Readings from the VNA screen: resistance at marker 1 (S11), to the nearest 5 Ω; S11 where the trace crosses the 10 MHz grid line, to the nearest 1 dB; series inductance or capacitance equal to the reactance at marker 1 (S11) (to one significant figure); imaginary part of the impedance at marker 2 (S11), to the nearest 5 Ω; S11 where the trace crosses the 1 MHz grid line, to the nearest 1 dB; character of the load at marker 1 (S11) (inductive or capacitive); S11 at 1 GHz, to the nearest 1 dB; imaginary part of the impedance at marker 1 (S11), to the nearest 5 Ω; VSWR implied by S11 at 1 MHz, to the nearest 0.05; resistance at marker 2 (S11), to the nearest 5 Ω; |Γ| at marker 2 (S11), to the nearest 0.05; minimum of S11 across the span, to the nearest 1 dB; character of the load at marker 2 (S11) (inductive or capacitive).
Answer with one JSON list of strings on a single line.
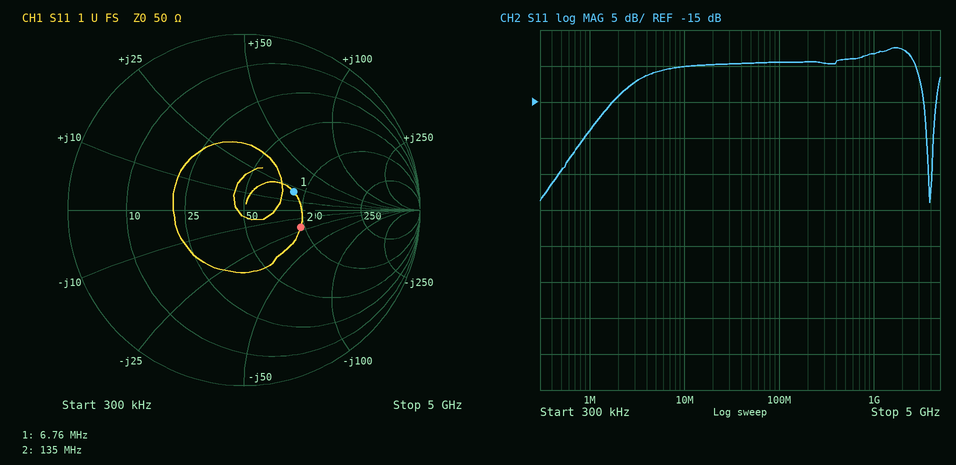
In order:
["85 Ω", "-10 dB", "500 nH", "-20 Ω", "-19 dB", "inductive", "-8 dB", "+20 Ω", "1.25", "95 Ω", "0.35", "-29 dB", "capacitive"]
